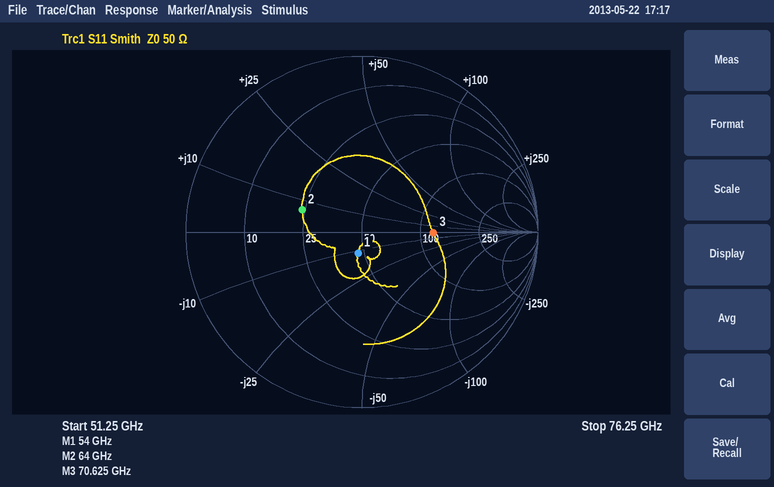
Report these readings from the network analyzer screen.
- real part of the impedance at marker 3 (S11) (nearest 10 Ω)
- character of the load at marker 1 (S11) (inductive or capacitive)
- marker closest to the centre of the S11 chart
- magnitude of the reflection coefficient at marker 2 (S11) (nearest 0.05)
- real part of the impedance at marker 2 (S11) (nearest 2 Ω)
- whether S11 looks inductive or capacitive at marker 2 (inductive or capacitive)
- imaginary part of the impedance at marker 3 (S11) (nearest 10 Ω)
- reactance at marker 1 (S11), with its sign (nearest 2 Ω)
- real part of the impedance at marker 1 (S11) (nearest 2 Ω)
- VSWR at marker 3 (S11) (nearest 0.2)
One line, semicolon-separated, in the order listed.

120 Ω; capacitive; marker 1; 0.35; 24 Ω; inductive; 0 Ω; -12 Ω; 46 Ω; 2.4
